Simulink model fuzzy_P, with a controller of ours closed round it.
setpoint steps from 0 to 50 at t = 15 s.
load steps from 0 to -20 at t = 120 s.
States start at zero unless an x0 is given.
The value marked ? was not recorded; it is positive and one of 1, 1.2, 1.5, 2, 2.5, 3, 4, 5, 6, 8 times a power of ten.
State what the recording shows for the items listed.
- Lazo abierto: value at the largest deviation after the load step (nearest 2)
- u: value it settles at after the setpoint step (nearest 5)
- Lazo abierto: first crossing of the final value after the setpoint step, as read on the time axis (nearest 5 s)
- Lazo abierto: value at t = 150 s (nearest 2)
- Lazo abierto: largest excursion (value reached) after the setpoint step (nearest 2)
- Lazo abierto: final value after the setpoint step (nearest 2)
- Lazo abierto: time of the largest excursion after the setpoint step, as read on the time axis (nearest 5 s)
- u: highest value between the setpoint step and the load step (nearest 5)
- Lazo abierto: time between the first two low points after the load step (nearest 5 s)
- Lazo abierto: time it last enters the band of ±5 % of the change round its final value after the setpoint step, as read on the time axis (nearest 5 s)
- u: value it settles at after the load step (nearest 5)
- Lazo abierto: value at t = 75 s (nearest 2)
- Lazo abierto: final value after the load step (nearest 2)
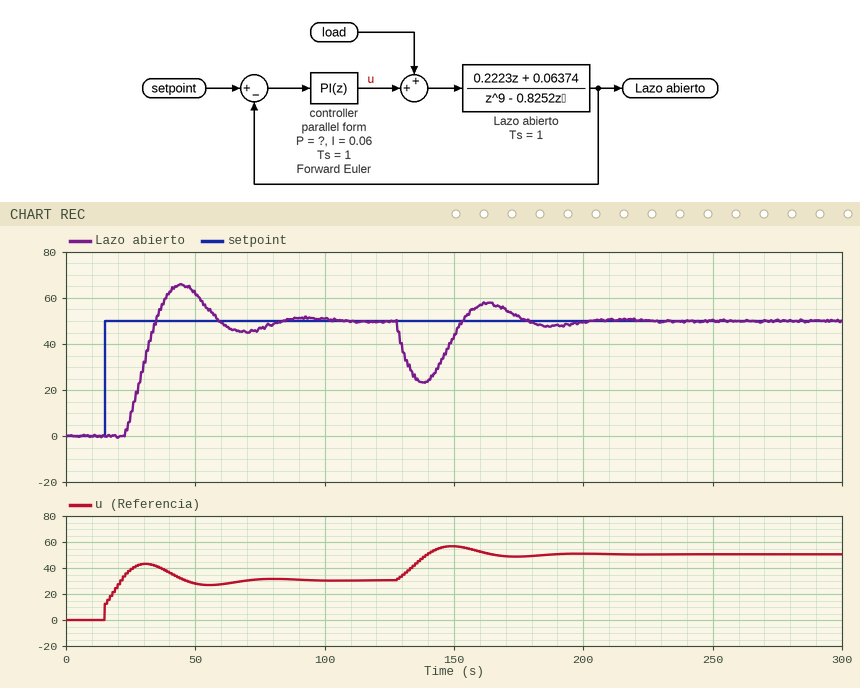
24
30
35 s
44
66
50
45 s
45
50 s
75 s
50
46
50
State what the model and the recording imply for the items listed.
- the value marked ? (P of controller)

0.25
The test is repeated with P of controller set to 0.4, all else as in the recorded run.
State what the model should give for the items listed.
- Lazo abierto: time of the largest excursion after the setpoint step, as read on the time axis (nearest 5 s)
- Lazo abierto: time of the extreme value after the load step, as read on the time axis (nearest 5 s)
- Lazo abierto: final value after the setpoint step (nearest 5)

40 s
135 s
50
